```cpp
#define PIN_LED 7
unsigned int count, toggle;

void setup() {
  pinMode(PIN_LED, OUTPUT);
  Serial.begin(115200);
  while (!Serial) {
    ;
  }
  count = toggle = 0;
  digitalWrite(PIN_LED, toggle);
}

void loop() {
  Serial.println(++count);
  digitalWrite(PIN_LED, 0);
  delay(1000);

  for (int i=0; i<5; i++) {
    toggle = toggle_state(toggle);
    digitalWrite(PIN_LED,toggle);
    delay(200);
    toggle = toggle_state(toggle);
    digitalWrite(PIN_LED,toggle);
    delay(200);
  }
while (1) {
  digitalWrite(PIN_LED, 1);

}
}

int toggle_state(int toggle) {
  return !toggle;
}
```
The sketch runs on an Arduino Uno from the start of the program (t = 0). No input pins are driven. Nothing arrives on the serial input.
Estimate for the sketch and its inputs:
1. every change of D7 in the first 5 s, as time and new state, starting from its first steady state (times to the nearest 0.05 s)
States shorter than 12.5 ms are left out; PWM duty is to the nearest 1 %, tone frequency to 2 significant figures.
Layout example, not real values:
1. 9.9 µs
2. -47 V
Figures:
1. 0 s low; 1 s high; 1.2 s low; 1.4 s high; 1.6 s low; 1.8 s high; 2 s low; 2.2 s high; 2.4 s low; 2.6 s high; 2.8 s low; 3 s high
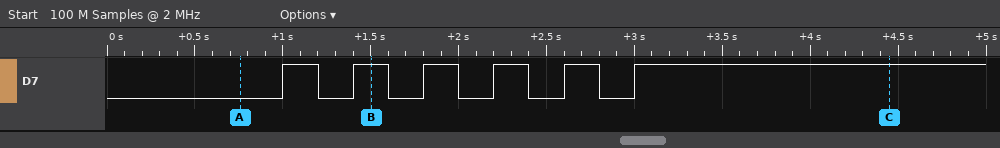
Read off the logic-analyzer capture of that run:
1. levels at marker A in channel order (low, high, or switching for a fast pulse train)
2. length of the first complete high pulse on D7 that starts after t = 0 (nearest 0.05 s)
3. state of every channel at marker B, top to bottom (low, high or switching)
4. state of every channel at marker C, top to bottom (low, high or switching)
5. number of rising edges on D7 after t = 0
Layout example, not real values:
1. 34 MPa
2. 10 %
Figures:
1. D7 low
2. 0.20 s
3. D7 high
4. D7 high
5. 6
